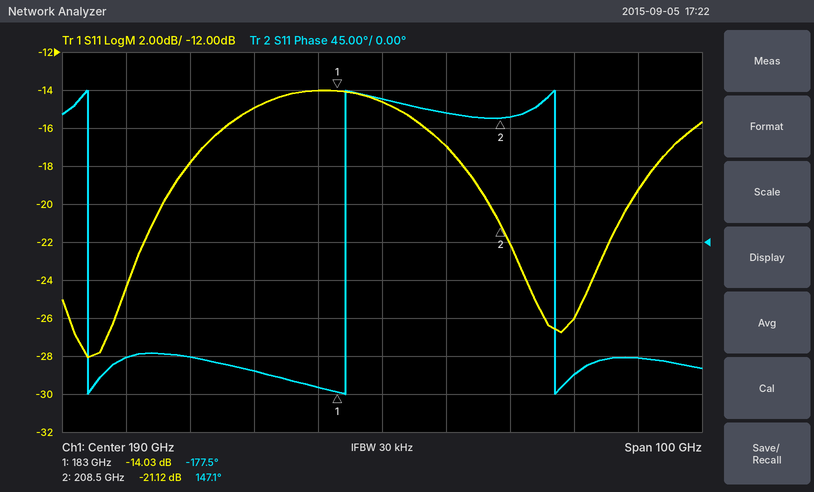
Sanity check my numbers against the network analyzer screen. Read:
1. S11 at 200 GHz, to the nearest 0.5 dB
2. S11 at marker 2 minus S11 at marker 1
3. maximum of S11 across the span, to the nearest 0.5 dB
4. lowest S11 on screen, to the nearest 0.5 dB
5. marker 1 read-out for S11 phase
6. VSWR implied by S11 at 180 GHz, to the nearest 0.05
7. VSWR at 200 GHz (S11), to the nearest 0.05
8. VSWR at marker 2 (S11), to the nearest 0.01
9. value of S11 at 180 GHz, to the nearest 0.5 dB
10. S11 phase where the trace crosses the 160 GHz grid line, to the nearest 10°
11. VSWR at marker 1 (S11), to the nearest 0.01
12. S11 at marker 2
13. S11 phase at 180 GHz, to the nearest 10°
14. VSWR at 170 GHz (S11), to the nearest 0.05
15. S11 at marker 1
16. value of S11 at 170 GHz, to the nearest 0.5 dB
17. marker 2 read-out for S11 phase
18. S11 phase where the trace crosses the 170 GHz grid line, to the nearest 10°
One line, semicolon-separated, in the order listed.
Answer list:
-17.0 dB; -7.09 dB; -14.0 dB; -28.0 dB; -177.5°; 1.50; 1.35; 1.19; -14.0 dB; -140°; 1.50; -21.12 dB; -170°; 1.45; -14.03 dB; -15.0 dB; 147.1°; -150°
